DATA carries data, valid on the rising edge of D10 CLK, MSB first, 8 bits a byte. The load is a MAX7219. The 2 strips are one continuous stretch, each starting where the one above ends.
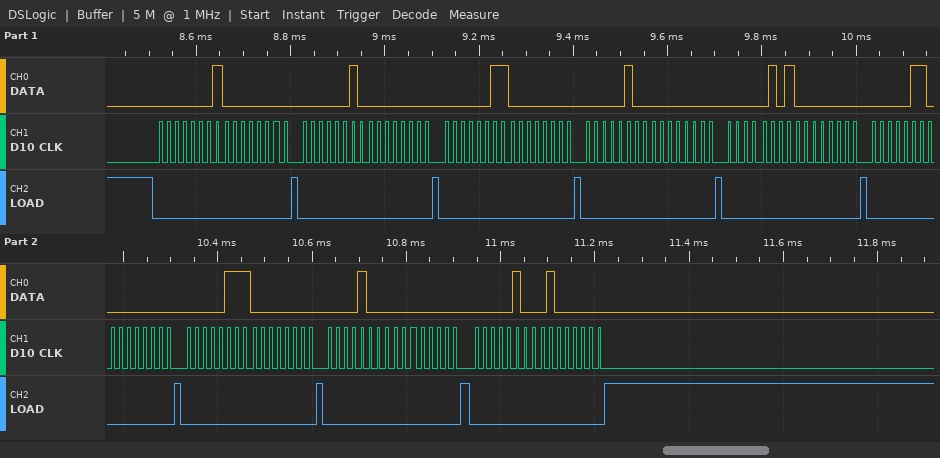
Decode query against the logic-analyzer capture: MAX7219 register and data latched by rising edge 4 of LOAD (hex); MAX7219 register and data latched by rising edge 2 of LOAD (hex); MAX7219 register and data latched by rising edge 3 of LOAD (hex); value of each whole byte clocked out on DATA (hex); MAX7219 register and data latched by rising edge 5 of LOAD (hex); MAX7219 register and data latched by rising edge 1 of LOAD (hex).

register 0x4, data 0x00
register 0x2, data 0x00
register 0x3, data 0x00
01 00 02 00 03 00 04 00 05 00 06 00 07 00 08 00 04 40
register 0x5, data 0x00
register 0x1, data 0x00
